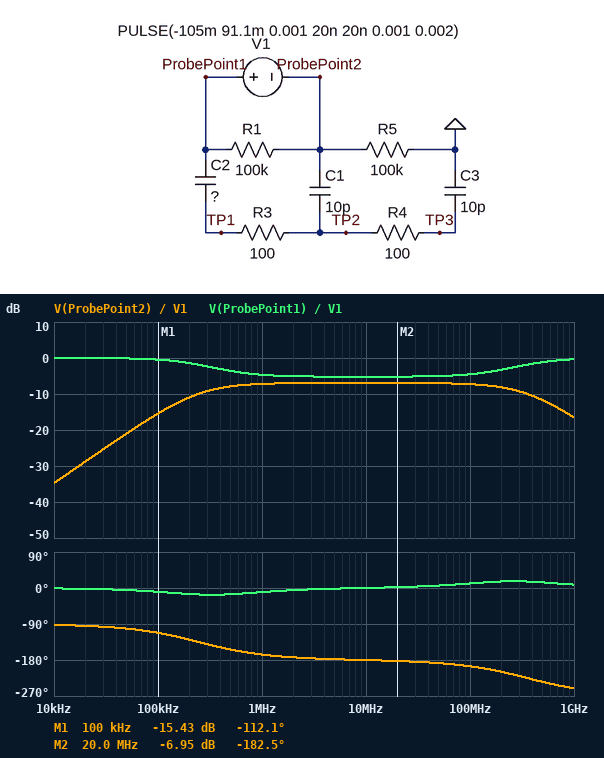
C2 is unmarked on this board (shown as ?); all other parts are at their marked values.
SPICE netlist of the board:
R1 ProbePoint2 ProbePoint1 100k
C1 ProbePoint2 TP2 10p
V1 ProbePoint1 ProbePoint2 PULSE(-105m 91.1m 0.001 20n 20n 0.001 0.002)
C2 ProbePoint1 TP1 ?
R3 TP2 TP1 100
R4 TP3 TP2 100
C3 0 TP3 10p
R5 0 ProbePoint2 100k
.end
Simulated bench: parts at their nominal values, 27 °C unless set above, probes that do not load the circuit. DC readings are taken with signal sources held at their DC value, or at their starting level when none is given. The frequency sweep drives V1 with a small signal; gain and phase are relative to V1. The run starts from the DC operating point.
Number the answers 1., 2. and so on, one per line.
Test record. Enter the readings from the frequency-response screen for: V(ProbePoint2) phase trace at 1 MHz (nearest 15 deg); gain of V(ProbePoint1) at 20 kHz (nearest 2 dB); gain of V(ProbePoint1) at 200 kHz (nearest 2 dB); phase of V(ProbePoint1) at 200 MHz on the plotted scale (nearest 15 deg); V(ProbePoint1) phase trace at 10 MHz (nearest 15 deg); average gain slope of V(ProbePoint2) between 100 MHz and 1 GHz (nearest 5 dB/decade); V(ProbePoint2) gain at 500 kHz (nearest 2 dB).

1. -165 deg
2. 0 dB
3. -2 dB
4. 15 deg
5. 0 deg
6. -10 dB/decade
7. -8 dB
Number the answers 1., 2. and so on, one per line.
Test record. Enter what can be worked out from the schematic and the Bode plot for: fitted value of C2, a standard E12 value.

1. 8.2 pF
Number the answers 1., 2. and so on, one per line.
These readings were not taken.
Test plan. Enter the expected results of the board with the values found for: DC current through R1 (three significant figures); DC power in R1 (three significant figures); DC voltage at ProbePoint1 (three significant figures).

1. 1.05 µA
2. 110 nW
3. -105 mV
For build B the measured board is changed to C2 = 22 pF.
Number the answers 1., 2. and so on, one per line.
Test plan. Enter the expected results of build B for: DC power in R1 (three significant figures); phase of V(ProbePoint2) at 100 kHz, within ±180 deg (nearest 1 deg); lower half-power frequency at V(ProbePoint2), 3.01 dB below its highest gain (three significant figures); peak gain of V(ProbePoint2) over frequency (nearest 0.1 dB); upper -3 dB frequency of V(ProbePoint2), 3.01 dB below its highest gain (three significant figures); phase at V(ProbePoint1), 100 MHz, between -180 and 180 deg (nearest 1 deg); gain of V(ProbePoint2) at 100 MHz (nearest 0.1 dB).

1. 110 nW
2. -116 deg
3. 208 kHz
4. -3.3 dB
5. 232 MHz
6. 31 deg
7. -4.0 dB
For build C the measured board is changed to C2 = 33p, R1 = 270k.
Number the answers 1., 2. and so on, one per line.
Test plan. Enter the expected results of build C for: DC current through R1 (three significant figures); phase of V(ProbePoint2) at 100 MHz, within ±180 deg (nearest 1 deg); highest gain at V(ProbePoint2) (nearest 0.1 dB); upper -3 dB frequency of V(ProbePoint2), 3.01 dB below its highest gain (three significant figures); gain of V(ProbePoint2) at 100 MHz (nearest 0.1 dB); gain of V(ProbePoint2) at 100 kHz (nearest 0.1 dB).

1. 389 nA
2. 154 deg
3. -2.3 dB
4. 208 MHz
5. -3.2 dB
6. -9.2 dB
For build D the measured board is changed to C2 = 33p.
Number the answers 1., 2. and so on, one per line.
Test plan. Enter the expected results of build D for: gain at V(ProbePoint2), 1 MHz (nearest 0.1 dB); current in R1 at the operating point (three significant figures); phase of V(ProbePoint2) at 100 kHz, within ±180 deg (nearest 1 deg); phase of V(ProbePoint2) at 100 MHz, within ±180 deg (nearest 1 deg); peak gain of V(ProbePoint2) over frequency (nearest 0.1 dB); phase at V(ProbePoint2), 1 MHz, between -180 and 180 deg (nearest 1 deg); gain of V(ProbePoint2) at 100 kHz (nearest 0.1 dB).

1. -2.5 dB
2. 1.05 µA
3. -117 deg
4. 154 deg
5. -2.3 dB
6. -169 deg
7. -9.2 dB
